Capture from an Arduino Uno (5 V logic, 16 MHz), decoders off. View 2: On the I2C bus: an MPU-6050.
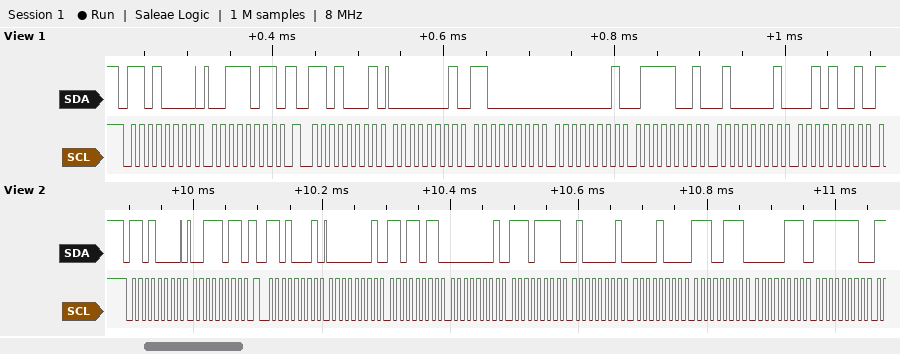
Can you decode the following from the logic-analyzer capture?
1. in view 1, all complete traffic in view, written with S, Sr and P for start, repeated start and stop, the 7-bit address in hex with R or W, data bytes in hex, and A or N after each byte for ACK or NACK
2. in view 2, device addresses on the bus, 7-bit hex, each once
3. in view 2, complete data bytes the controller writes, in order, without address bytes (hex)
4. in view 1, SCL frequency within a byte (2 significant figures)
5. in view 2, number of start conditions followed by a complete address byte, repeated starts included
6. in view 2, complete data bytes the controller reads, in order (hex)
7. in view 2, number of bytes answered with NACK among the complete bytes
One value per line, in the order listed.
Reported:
S 68W A 3B A Sr 68R A 01 A C0 A 01 A 79 A 41 A 29 A
0x68
3B
100 kHz
2
01 DB 01 EF 41 08 E7 07 FE
0
